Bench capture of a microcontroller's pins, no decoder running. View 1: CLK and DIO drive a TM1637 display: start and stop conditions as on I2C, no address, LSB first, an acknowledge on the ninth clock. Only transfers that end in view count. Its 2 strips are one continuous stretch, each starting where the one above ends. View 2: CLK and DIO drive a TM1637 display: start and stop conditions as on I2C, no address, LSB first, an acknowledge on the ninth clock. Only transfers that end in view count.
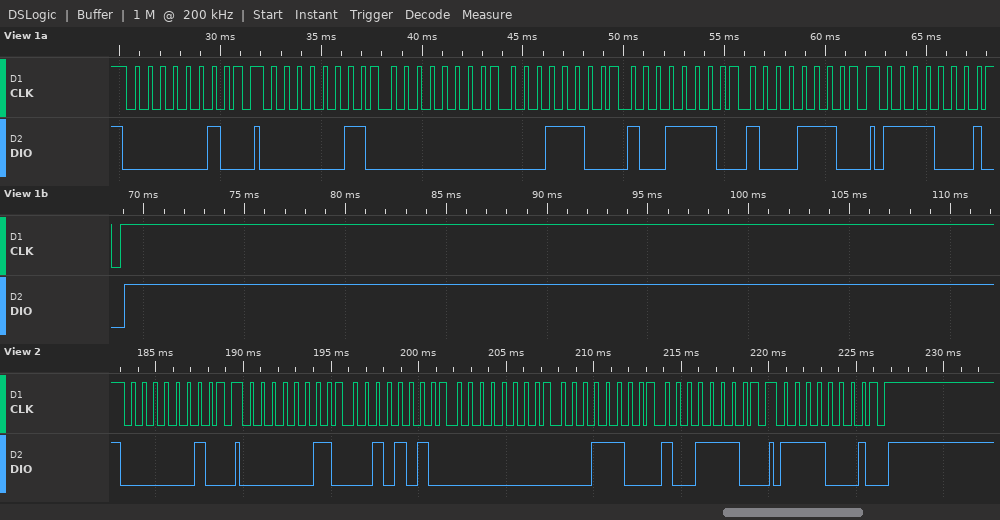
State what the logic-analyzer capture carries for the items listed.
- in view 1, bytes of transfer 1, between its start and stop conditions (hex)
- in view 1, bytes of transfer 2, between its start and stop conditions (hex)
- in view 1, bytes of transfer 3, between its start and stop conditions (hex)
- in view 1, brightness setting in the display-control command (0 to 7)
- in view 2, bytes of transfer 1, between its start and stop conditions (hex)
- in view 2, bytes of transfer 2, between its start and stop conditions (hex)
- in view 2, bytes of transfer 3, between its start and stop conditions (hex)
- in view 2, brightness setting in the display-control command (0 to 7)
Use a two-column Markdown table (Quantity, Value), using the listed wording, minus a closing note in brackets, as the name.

| Quantity | Value |
|---|---|
| in view 1, bytes of transfer 1, between its start and stop conditions | 40 |
| in view 1, bytes of transfer 2, between its start and stop conditions | C0 00 38 79 71 |
| in view 1, bytes of transfer 3, between its start and stop conditions | 8F |
| in view 1, brightness setting in the display-control command | 7 |
| in view 2, bytes of transfer 1, between its start and stop conditions | 40 |
| in view 2, bytes of transfer 2, between its start and stop conditions | C0 54 00 38 79 |
| in view 2, bytes of transfer 3, between its start and stop conditions | 8F |
| in view 2, brightness setting in the display-control command | 7 |
